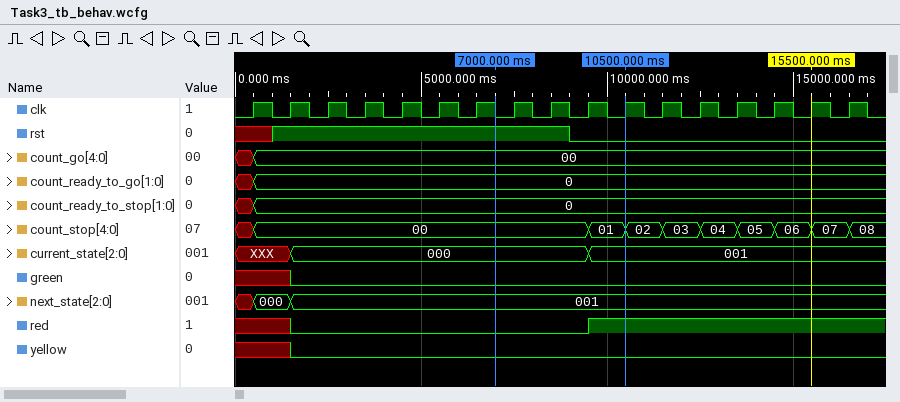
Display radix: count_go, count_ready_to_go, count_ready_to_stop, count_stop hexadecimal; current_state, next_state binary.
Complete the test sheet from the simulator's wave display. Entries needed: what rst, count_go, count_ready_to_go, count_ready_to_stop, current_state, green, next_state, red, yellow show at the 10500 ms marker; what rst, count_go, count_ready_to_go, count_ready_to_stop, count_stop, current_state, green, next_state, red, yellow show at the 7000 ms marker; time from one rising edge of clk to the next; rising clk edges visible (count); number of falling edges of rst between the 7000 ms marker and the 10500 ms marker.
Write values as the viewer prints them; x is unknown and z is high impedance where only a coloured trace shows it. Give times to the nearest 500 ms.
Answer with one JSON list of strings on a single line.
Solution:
["rst=0, count_go=00, count_ready_to_go=0, count_ready_to_stop=0, current_state=001, green=0, next_state=001, red=1, yellow=0", "rst=1, count_go=00, count_ready_to_go=0, count_ready_to_stop=0, count_stop=00, current_state=000, green=0, next_state=001, red=0, yellow=0", "1000 ms", "17", "1"]
